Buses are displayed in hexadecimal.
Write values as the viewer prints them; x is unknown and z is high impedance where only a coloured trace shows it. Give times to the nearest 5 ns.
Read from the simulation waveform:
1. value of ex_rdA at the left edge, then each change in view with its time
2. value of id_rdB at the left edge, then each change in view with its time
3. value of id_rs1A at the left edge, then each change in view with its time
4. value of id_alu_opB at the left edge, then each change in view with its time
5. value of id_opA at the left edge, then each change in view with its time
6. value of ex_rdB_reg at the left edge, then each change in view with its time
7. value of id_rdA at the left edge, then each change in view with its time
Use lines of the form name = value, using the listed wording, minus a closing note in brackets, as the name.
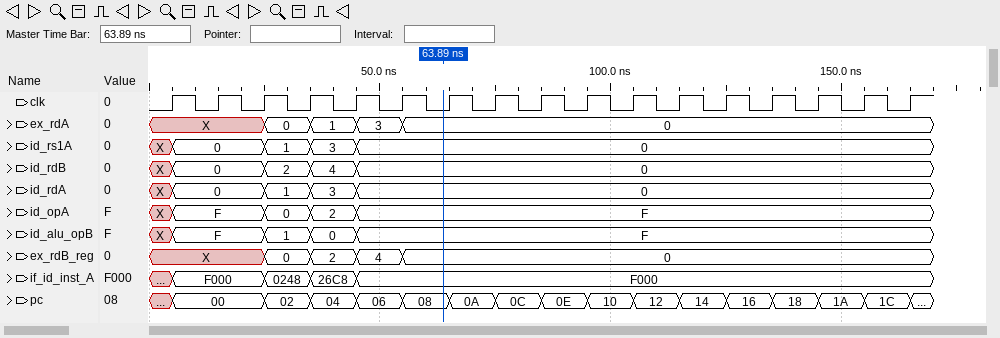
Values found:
value of ex_rdA at the left edge, then each change in view with its time = X, 0 at 25 ns, 1 at 35 ns, 3 at 45 ns, 0 at 55 ns
value of id_rdB at the left edge, then each change in view with its time = X, 0 at 5 ns, 2 at 25 ns, 4 at 35 ns, 0 at 45 ns
value of id_rs1A at the left edge, then each change in view with its time = X, 0 at 5 ns, 1 at 25 ns, 3 at 35 ns, 0 at 45 ns
value of id_alu_opB at the left edge, then each change in view with its time = X, F at 5 ns, 1 at 25 ns, 0 at 35 ns, F at 45 ns
value of id_opA at the left edge, then each change in view with its time = X, F at 5 ns, 0 at 25 ns, 2 at 35 ns, F at 45 ns
value of ex_rdB_reg at the left edge, then each change in view with its time = X, 0 at 25 ns, 2 at 35 ns, 4 at 45 ns, 0 at 55 ns
value of id_rdA at the left edge, then each change in view with its time = X, 0 at 5 ns, 1 at 25 ns, 3 at 35 ns, 0 at 45 ns
